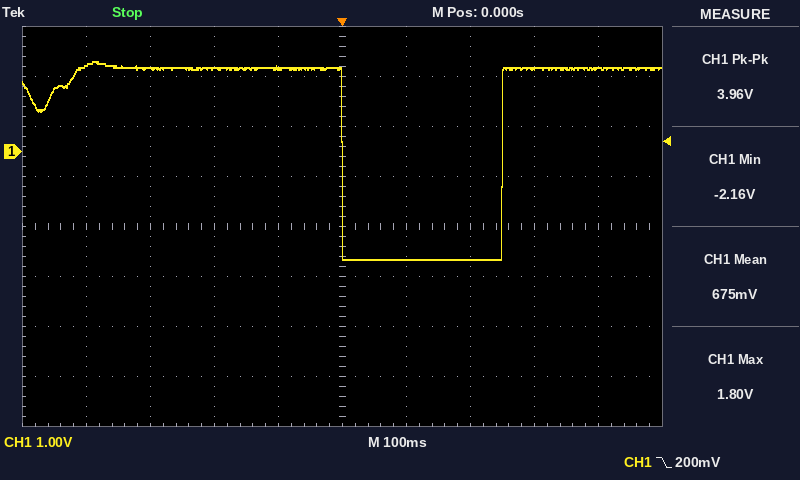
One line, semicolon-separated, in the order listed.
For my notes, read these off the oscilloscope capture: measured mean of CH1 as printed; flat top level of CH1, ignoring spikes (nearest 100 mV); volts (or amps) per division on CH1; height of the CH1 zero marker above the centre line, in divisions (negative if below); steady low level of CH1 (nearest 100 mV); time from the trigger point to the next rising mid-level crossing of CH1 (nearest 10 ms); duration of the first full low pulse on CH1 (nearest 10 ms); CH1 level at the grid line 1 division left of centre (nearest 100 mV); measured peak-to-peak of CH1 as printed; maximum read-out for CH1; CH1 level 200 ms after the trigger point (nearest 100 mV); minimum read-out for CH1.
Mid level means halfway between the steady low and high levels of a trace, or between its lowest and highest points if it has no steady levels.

675 mV; 1.7 V; 1 V; +1.5 div; -2.2 V; 250 ms; 250 ms; 1.7 V; 3.96 V; 1.80 V; -2.2 V; -2.16 V
